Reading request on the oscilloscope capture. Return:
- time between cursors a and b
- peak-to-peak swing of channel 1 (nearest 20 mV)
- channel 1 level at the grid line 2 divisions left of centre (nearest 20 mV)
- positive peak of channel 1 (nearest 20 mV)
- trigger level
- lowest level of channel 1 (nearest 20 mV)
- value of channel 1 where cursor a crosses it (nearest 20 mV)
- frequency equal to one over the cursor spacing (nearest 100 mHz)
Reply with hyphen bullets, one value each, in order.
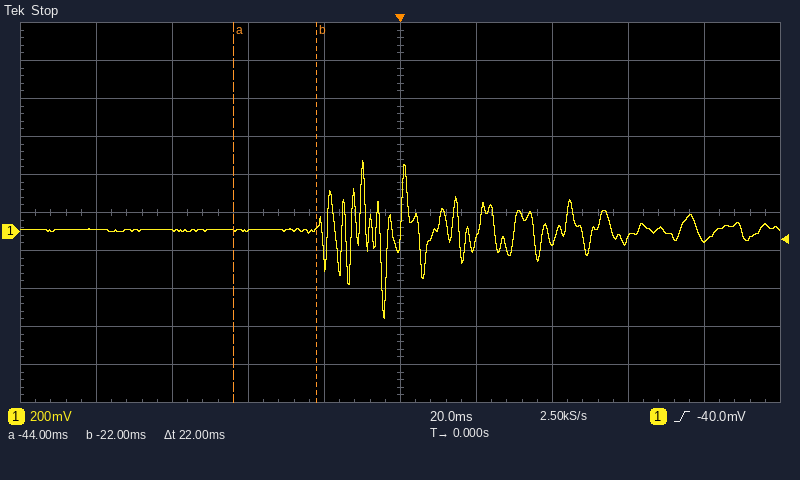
- 22 ms
- 840 mV
- 0 mV
- 380 mV
- -40.0 mV
- -460 mV
- 0 mV
- 45.5 Hz
